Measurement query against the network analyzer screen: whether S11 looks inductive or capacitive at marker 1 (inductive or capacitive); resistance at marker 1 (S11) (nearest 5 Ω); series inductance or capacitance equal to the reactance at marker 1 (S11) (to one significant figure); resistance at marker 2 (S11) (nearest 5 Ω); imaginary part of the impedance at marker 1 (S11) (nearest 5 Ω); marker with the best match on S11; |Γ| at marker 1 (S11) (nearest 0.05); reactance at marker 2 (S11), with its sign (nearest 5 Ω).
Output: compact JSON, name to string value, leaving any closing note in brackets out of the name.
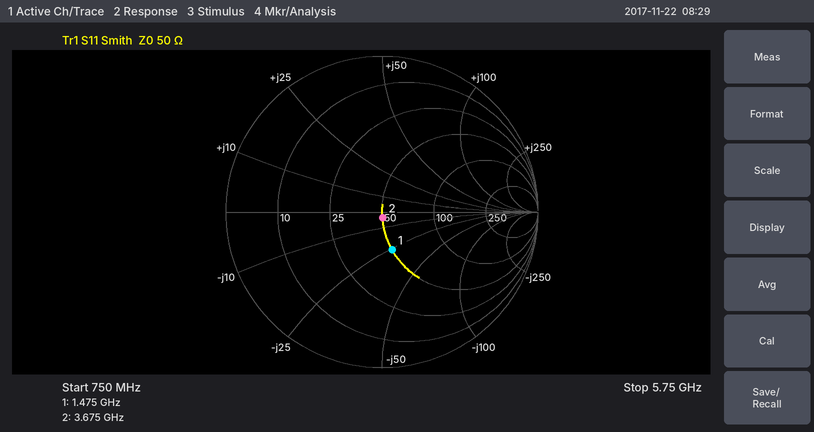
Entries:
{"whether S11 looks inductive or capacitive at marker 1": "capacitive", "resistance at marker 1 (S11)": "50 Ω", "series inductance or capacitance equal to the reactance at marker 1 (S11)": "4 pF", "resistance at marker 2 (S11)": "50 Ω", "imaginary part of the impedance at marker 1 (S11)": "-25 Ω", "marker with the best match on S11": "marker 2", "|Γ| at marker 1 (S11)": "0.25", "reactance at marker 2 (S11), with its sign": "-5 Ω"}
